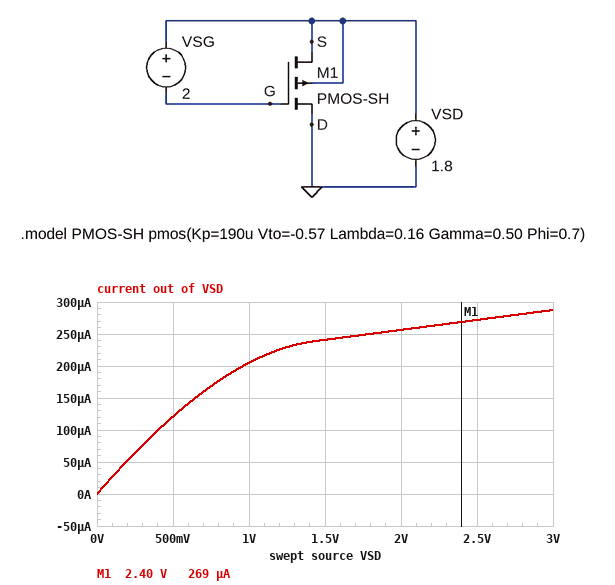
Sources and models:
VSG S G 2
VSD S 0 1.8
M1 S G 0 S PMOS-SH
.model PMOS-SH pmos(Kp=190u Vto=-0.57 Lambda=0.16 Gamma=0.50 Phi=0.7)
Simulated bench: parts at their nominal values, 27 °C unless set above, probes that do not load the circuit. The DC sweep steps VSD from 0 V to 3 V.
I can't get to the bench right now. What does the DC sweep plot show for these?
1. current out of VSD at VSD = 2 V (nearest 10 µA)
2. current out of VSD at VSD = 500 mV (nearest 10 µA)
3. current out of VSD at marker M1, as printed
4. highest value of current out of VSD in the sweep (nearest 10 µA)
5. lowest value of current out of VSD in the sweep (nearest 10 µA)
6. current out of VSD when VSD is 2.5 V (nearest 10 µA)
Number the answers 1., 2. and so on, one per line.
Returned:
1. 260 µA
2. 120 µA
3. 269 µA
4. 290 µA
5. 0 A
6. 270 µA
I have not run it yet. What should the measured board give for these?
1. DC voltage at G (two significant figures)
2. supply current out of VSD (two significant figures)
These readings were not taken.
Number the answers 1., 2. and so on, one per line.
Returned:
1. -200 mV
2. 250 µA
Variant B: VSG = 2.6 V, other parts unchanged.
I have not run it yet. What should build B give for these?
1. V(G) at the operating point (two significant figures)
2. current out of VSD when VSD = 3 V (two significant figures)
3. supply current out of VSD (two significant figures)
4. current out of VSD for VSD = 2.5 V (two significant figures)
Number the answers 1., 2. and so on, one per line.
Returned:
1. -800 mV
2. 580 µA
3. 500 µA
4. 550 µA
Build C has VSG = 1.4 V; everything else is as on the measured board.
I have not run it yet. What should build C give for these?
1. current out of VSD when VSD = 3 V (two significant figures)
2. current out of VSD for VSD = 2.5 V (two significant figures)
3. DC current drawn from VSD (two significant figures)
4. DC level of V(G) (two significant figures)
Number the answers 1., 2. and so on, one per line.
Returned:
1. 97 µA
2. 92 µA
3. 84 µA
4. 400 mV
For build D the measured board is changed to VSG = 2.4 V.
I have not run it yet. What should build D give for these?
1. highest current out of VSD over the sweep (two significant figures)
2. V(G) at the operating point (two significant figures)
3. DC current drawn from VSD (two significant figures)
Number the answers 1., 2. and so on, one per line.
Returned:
1. 470 µA
2. -600 mV
3. 410 µA
